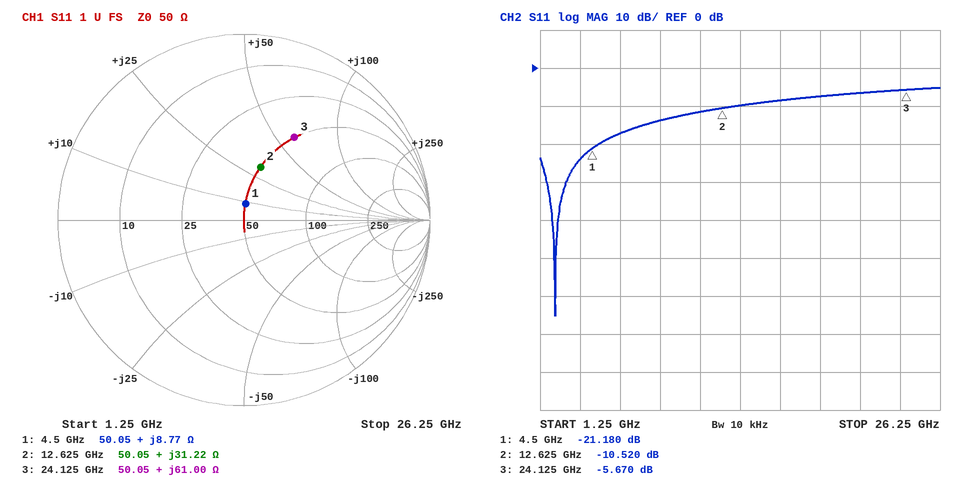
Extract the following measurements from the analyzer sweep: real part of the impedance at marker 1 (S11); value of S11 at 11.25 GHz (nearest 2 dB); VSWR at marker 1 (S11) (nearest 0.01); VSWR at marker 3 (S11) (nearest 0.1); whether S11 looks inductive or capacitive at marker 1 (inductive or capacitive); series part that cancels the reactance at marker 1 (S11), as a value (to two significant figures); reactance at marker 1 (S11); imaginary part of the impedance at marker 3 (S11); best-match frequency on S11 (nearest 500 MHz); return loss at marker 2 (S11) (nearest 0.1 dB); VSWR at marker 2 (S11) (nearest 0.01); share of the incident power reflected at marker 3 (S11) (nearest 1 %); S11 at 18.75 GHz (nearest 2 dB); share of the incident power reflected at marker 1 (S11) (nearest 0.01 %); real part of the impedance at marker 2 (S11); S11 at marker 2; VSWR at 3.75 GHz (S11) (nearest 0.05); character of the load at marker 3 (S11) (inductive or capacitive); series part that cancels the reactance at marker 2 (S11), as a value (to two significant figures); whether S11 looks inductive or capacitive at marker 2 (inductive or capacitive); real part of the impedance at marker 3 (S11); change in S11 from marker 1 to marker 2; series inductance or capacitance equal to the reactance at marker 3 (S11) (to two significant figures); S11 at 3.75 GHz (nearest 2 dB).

50.05 Ω
-12 dB
1.19
3.2
inductive
4.0 pF
+8.77 Ω
+61.00 Ω
2.0 GHz
10.5 dB
1.85
27 %
-8 dB
0.76 %
50.05 Ω
-10.520 dB
1.15
inductive
400 fF
inductive
50.05 Ω
10.660 dB
400 pH
-24 dB
